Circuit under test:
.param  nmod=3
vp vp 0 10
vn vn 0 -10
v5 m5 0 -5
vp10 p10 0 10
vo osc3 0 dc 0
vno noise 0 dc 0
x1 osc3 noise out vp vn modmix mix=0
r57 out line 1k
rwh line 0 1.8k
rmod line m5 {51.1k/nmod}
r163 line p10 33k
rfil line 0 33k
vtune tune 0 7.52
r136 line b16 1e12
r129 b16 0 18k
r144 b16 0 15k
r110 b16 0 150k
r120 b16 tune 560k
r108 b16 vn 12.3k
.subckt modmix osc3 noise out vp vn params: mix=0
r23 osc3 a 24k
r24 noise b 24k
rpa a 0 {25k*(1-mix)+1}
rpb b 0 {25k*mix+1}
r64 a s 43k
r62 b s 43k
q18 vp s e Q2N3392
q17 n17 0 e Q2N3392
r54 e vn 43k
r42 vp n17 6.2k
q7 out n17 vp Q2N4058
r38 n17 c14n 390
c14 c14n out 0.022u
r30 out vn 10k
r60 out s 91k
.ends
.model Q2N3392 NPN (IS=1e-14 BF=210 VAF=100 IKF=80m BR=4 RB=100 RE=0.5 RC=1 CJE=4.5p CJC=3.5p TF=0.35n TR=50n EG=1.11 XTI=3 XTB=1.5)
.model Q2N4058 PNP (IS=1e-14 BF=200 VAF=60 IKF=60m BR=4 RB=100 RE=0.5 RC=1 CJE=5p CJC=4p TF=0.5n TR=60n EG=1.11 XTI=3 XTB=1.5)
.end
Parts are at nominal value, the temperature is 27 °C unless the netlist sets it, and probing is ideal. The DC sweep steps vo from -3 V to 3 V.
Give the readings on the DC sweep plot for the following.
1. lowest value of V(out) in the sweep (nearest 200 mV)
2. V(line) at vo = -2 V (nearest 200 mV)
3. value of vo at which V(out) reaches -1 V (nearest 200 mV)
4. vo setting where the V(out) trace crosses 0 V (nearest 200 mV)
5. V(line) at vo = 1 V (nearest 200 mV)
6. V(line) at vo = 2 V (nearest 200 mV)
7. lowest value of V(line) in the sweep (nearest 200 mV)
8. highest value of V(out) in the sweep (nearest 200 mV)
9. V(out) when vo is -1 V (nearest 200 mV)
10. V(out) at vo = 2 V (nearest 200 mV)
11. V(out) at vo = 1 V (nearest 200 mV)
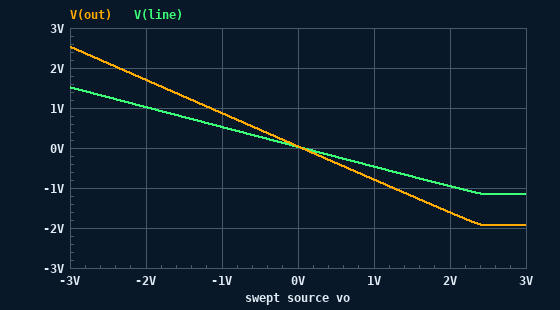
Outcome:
-2.0 V
1.0 V
1.2 V
0 V
-400 mV
-1.0 V
-1.2 V
2.6 V
800 mV
-1.6 V
-800 mV
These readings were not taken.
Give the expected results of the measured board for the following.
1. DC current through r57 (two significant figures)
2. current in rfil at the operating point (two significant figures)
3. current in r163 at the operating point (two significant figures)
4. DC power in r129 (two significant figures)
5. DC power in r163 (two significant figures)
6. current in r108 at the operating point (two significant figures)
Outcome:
10 µA
890 nA
300 µA
790 µW
3.0 mW
510 µA
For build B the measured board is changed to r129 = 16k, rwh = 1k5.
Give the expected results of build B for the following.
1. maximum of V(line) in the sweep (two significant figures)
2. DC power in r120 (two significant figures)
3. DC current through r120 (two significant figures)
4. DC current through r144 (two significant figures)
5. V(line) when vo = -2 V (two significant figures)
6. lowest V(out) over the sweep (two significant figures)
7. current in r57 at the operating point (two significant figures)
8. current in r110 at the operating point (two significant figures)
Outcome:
1.4 V
220 µW
20 µA
240 µA
960 mV
-1.8 V
12 µA
24 µA
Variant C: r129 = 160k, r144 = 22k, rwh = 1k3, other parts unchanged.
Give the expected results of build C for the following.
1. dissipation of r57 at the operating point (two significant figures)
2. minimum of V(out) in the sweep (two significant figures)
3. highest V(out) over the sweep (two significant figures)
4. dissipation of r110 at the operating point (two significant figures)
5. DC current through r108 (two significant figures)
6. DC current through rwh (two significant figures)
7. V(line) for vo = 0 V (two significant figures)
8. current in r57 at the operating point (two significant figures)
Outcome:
190 nW
-1.7 V
2.5 V
210 µW
350 µA
20 µA
26 mV
14 µA
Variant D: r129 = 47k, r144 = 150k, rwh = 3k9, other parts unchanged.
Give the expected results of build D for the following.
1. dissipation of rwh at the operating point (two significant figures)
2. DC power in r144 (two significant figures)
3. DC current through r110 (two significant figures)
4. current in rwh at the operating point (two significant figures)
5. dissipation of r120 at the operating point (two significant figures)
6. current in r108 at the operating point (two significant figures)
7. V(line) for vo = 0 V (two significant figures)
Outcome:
330 nW
310 µW
45 µA
9.2 µA
370 µW
260 µA
36 mV
